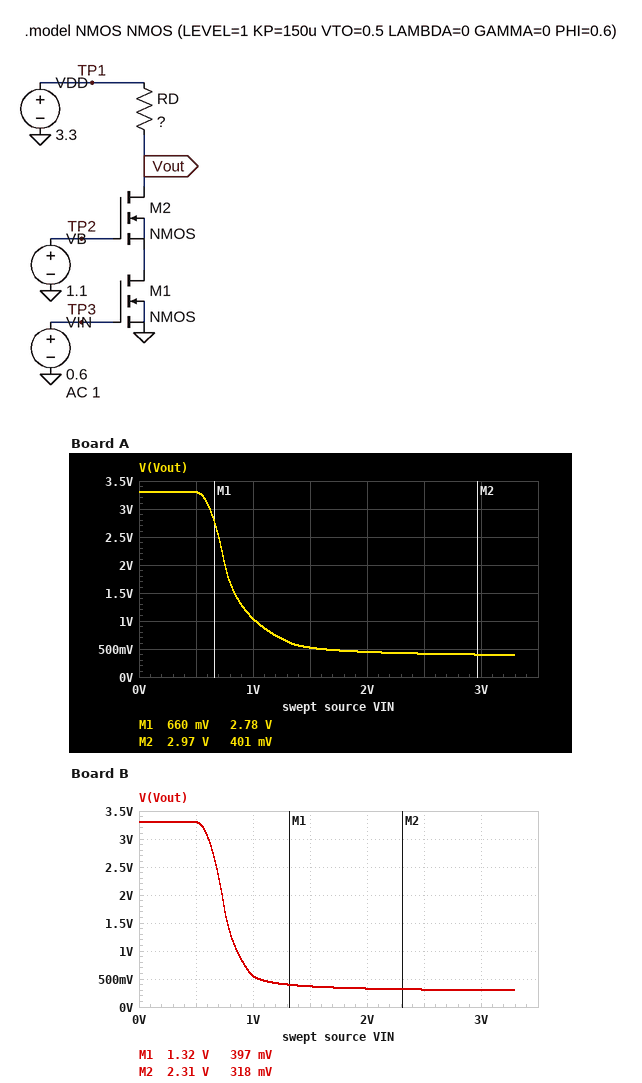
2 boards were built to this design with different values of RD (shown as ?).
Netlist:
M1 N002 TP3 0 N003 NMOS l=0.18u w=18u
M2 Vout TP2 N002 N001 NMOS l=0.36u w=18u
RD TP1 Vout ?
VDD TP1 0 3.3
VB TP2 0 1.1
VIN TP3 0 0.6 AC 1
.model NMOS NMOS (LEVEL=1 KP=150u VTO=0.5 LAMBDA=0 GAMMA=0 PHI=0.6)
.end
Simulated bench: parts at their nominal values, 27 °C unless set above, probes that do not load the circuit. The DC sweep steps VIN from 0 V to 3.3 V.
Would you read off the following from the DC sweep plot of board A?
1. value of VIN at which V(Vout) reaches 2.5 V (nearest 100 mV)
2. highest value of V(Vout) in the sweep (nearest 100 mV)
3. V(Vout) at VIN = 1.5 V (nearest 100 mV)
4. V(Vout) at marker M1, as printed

700 mV
3.3 V
500 mV
2.78 V
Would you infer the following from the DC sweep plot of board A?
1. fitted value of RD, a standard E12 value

2.7 kΩ
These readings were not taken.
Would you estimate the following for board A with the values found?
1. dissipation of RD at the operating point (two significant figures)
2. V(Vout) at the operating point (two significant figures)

15 µW
3.1 V
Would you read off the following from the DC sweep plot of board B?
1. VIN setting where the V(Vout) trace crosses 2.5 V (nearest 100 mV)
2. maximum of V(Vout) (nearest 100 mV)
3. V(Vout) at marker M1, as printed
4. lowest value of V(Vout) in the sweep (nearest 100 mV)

700 mV
3.3 V
397 mV
300 mV
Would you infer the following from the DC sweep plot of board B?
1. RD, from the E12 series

3.3 kΩ
